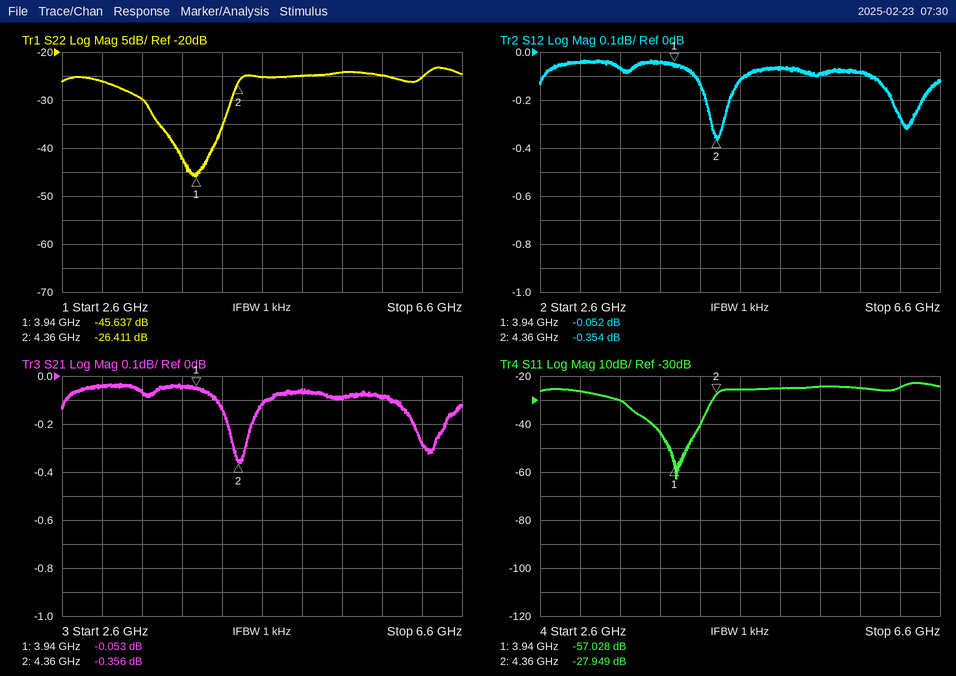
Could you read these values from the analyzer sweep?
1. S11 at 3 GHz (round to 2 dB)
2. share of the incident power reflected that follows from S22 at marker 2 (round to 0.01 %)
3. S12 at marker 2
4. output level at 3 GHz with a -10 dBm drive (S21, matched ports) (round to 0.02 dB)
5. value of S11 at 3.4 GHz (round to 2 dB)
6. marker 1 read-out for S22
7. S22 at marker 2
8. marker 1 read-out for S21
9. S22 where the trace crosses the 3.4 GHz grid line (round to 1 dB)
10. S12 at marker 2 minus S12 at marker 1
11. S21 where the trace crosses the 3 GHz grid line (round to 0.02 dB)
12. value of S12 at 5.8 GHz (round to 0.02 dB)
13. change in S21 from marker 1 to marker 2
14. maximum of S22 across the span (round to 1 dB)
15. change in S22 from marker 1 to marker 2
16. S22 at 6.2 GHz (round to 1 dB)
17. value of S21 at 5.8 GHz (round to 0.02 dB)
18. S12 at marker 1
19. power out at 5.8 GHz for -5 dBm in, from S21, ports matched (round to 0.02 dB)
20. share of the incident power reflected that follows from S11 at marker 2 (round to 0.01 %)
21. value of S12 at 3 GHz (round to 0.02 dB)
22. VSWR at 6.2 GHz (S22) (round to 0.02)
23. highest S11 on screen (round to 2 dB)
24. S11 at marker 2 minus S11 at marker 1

-26 dB
0.23 %
-0.354 dB
-10.04 dBm
-30 dB
-45.637 dB
-26.411 dB
-0.053 dB
-30 dB
-0.302 dB
-0.04 dB
-0.08 dB
-0.303 dB
-23 dB
19.226 dB
-25 dB
-0.08 dB
-0.052 dB
-5.08 dBm
0.16 %
-0.04 dB
1.12
-22 dB
29.079 dB
